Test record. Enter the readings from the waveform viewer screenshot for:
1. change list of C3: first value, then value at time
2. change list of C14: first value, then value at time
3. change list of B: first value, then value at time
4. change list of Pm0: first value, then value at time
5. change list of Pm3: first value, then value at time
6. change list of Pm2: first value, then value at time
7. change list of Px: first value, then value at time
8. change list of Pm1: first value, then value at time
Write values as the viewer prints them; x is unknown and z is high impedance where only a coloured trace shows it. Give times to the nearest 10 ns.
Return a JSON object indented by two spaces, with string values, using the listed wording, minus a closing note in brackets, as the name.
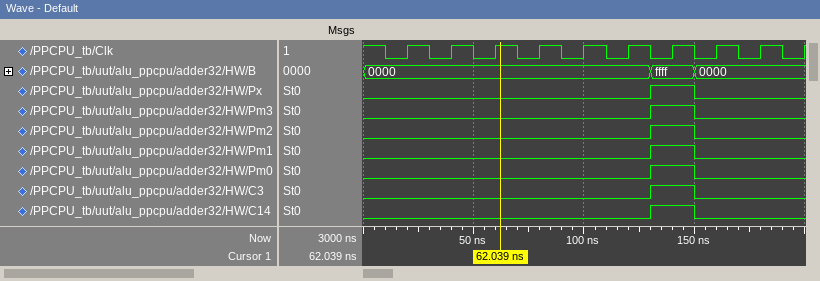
{
  "change list of C3: first value, then value at time": "0, 1 at 130 ns, 0 at 150 ns",
  "change list of C14: first value, then value at time": "0, 1 at 130 ns, 0 at 150 ns",
  "change list of B: first value, then value at time": "0000, ffff at 130 ns, 0000 at 150 ns",
  "change list of Pm0: first value, then value at time": "0, 1 at 130 ns, 0 at 150 ns",
  "change list of Pm3: first value, then value at time": "0, 1 at 130 ns, 0 at 150 ns",
  "change list of Pm2: first value, then value at time": "0, 1 at 130 ns, 0 at 150 ns",
  "change list of Px: first value, then value at time": "0, 1 at 130 ns, 0 at 150 ns",
  "change list of Pm1: first value, then value at time": "0, 1 at 130 ns, 0 at 150 ns"
}
